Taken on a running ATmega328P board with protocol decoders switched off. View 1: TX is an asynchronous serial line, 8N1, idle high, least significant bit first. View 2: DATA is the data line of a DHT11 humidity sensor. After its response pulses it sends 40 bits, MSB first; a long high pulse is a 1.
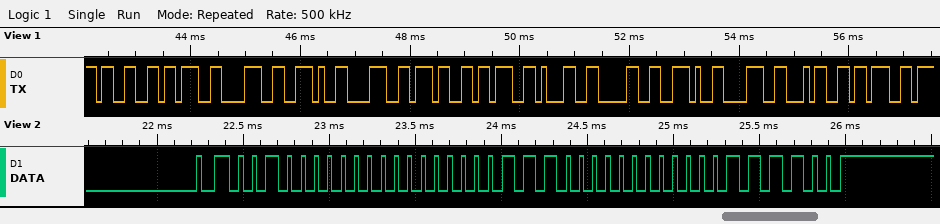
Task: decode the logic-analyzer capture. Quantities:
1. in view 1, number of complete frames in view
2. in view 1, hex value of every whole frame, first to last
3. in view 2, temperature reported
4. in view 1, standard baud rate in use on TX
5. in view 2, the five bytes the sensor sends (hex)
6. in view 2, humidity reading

13
33 3B 38 2E 38 37 3B 31 30 2E 38 34 3B
28.0 °C
9600 baud
20 00 1C 00 3C
32 %
